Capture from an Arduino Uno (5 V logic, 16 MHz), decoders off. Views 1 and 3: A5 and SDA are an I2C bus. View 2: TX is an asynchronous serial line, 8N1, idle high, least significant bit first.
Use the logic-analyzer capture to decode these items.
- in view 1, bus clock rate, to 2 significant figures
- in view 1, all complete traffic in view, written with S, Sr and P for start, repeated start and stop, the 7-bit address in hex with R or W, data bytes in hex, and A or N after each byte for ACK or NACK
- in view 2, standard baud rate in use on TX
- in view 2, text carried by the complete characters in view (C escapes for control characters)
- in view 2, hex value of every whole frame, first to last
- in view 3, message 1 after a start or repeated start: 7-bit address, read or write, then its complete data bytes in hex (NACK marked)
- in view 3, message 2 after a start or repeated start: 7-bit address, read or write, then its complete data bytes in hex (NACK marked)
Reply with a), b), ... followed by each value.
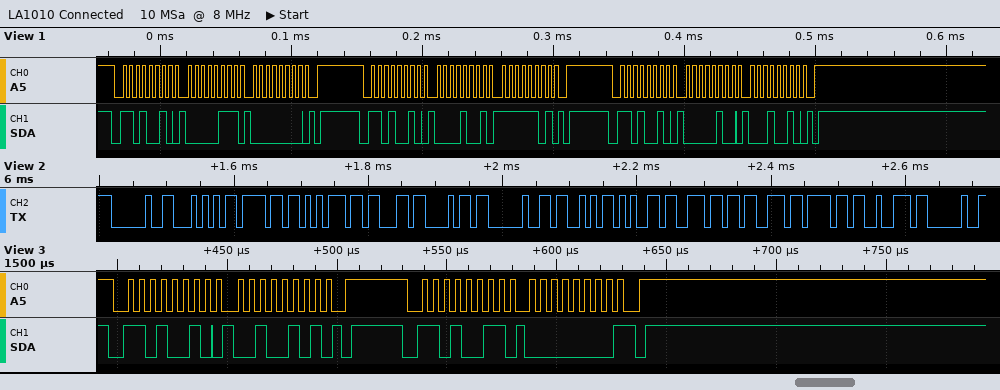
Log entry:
a) 200 kHz
b) S 69W A 07 A 00 A P S 69W A 09 A FD A P S 69W A 04 A 12 A P
c) 115200 baud
d) " Touch Sensor "
e) 20 54 6F 75 63 68 20 53 65 6E 73 6F 72 20
f) 0x69 write: 25
g) 0x69 read: 00 NACK
